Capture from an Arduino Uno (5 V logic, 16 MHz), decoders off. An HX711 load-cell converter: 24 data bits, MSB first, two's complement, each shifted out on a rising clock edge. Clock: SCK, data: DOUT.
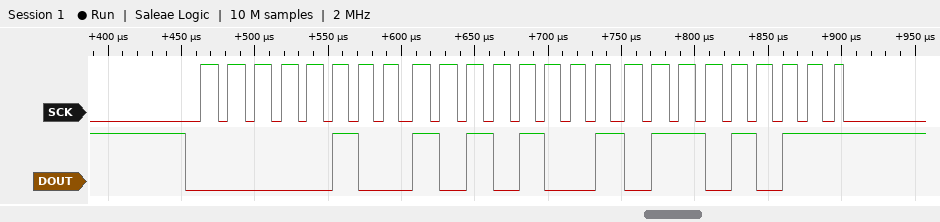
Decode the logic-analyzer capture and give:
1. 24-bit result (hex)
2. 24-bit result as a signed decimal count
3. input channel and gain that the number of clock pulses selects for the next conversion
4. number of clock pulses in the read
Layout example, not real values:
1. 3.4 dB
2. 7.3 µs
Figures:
1. 0x04A96B
2. 305515
3. channel A, gain 128
4. 25
